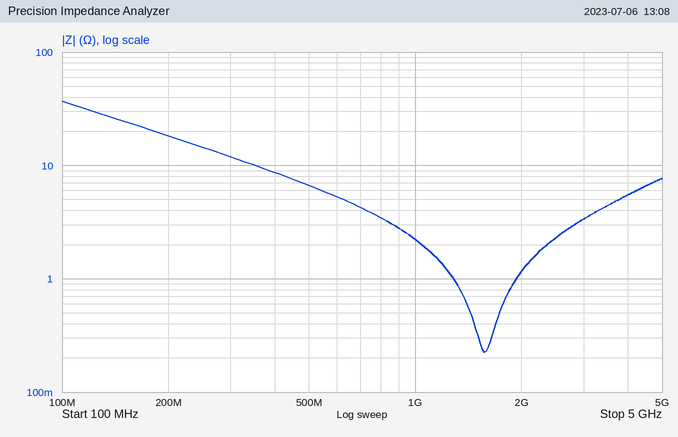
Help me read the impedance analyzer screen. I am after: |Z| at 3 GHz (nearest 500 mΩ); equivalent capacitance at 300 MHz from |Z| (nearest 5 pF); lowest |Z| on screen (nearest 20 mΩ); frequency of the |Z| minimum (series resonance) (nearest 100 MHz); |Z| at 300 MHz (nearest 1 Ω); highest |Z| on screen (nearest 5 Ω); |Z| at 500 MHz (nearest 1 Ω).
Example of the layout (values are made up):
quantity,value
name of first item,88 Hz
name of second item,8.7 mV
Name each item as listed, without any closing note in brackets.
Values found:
quantity,value
|Z| at 3 GHz,3.5 Ω
equivalent capacitance at 300 MHz from |Z|,45 pF
lowest |Z| on screen,220 mΩ
frequency of the |Z| minimum (series resonance),1.6 GHz
|Z| at 300 MHz,12 Ω
highest |Z| on screen,35 Ω
|Z| at 500 MHz,7 Ω
